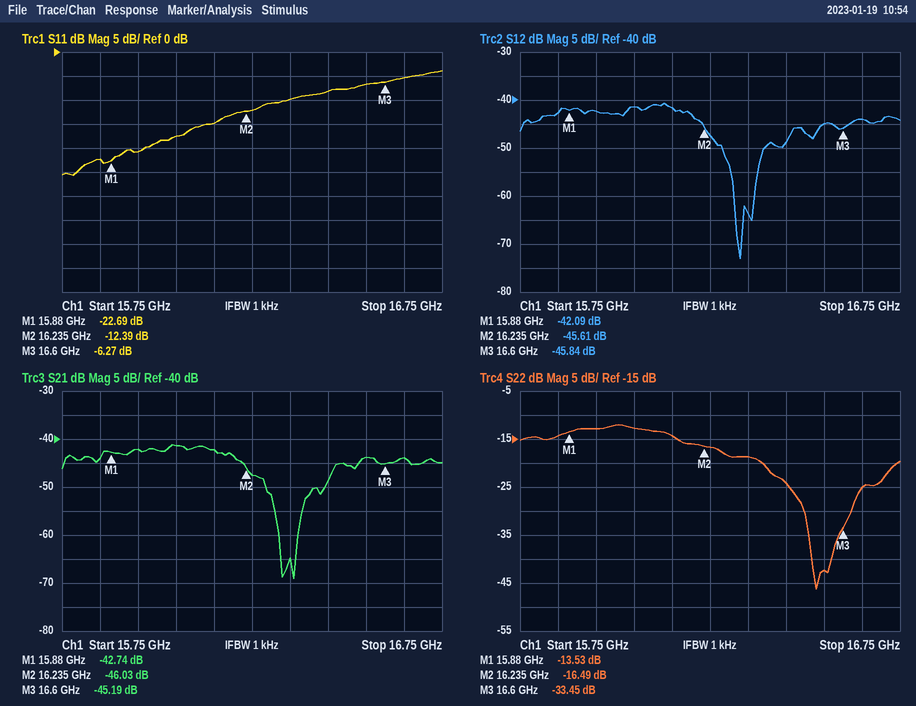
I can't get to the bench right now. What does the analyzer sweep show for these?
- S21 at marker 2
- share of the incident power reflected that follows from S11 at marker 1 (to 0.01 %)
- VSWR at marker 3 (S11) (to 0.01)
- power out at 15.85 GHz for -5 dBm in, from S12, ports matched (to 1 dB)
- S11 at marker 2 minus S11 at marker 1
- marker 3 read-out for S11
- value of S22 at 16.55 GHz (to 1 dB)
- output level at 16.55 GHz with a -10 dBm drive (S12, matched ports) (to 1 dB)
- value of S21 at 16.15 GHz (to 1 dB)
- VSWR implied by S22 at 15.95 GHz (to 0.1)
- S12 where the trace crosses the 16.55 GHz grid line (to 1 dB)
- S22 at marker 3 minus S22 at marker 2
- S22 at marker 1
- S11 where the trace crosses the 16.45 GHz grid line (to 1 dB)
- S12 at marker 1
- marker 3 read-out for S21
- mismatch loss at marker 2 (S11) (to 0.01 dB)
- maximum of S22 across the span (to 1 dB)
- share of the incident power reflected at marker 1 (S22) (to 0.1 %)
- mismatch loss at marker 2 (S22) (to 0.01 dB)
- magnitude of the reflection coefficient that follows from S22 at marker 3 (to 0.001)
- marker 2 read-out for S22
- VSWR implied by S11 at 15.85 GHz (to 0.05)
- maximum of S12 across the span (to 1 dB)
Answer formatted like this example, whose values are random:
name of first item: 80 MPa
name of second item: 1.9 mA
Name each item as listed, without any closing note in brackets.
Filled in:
S21 at marker 2: -46.03 dB
share of the incident power reflected that follows from S11 at marker 1: 0.54 %
VSWR at marker 3 (S11): 2.89
power out at 15.85 GHz for -5 dBm in, from S12, ports matched: -48 dBm
S11 at marker 2 minus S11 at marker 1: 10.30 dB
marker 3 read-out for S11: -6.27 dB
value of S22 at 16.55 GHz: -42 dB
output level at 16.55 GHz with a -10 dBm drive (S12, matched ports): -55 dBm
value of S21 at 16.15 GHz: -42 dB
VSWR implied by S22 at 15.95 GHz: 1.6
S12 where the trace crosses the 16.55 GHz grid line: -45 dB
S22 at marker 3 minus S22 at marker 2: -16.96 dB
S22 at marker 1: -13.53 dB
S11 where the trace crosses the 16.45 GHz grid line: -8 dB
S12 at marker 1: -42.09 dB
marker 3 read-out for S21: -45.19 dB
mismatch loss at marker 2 (S11): 0.26 dB
maximum of S22 across the span: -12 dB
share of the incident power reflected at marker 1 (S22): 4.4 %
mismatch loss at marker 2 (S22): 0.10 dB
magnitude of the reflection coefficient that follows from S22 at marker 3: 0.021
marker 2 read-out for S22: -16.49 dB
VSWR implied by S11 at 15.85 GHz: 1.15
maximum of S12 across the span: -41 dB
